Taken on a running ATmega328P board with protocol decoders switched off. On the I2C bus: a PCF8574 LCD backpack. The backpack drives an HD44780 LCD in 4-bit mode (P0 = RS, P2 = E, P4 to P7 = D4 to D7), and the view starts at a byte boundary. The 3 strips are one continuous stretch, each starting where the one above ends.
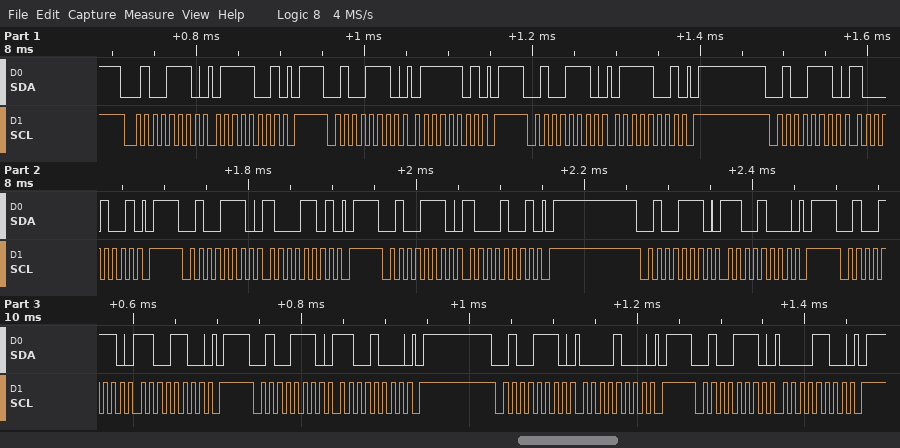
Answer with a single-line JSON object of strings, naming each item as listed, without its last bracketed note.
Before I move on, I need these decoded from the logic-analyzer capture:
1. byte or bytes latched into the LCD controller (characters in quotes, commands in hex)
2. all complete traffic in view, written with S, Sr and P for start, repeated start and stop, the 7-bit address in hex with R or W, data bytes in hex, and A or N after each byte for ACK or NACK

{"byte or bytes latched into the LCD controller": "'x'", "all complete traffic in view, written with S, Sr and P for start, repeated start and stop, the 7-bit address in hex with R or W, data bytes in hex, and A or N after each byte for ACK or NACK": "S 27W A 79 A P S 27W A 7D A P S 27W A 79 A P S 27W A 89 A P S 27W A 8D A P S 27W A 89 A P S 27W A C8 A P S 27W A CC A P S 27W A C8 A P S 27W A 08 A P S 27W A 0C A P"}
